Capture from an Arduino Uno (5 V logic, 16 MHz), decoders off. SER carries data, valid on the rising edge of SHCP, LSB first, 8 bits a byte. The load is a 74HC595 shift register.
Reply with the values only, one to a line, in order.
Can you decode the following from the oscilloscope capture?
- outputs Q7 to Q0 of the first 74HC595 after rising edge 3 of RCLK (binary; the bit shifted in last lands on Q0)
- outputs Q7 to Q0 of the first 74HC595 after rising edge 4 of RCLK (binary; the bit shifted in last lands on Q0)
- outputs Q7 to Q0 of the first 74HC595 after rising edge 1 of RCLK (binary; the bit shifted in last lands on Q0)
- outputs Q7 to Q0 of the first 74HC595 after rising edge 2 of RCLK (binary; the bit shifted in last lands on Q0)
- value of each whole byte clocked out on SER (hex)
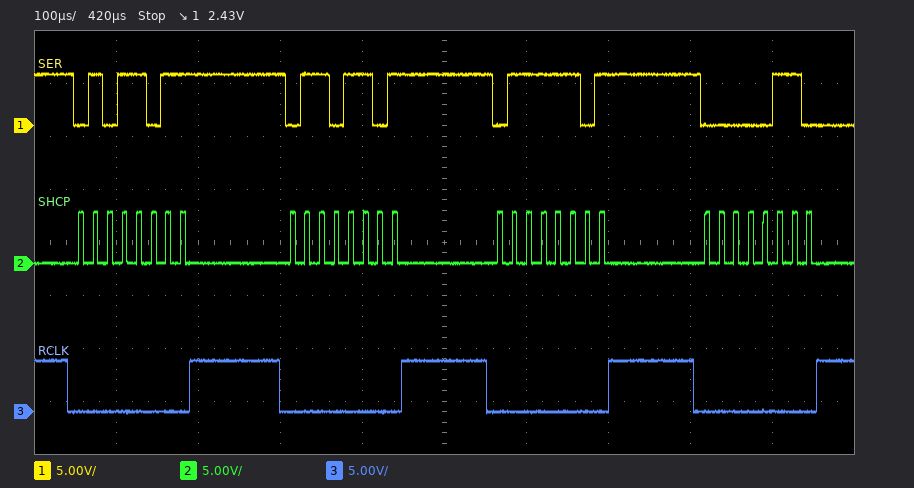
01111101
00000110
01011011
01101101
0xDA 0xB6 0xBE 0x60
